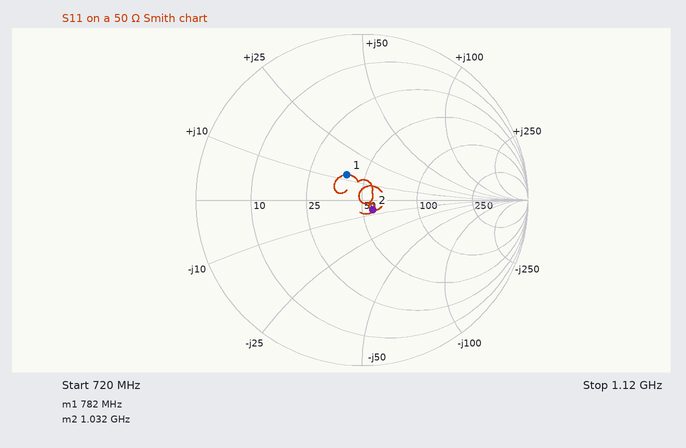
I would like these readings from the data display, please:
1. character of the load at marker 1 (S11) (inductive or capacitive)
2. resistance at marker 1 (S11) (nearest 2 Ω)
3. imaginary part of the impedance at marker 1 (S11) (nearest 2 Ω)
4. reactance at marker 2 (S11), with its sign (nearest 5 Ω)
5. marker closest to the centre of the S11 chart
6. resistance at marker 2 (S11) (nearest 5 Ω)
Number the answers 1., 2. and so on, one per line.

1. inductive
2. 40 Ω
3. +12 Ω
4. -5 Ω
5. marker 2
6. 55 Ω
